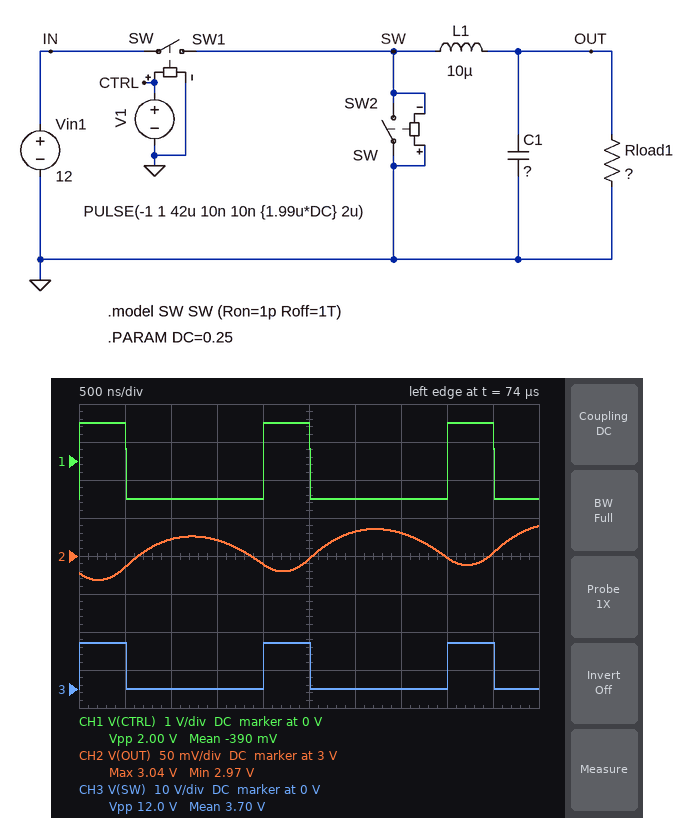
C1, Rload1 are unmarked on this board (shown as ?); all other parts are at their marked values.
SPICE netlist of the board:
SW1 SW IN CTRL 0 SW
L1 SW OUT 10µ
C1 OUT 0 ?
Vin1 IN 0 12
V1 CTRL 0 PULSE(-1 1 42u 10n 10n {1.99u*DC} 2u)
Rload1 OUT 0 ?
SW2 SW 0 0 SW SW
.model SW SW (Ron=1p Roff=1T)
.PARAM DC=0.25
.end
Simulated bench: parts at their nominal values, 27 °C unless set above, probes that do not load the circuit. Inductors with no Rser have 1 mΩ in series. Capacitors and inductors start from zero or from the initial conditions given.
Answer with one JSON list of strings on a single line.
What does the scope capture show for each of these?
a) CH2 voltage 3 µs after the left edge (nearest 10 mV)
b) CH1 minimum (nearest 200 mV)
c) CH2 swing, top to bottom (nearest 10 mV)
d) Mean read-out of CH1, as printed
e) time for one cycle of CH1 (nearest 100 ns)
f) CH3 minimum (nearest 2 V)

["3.03 V", "-1.0 V", "70 mV", "-390 mV", "2.0 µs", "0 V"]
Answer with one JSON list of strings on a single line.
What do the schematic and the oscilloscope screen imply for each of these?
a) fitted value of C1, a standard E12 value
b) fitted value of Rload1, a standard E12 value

["2.2 µF", "1 Ω"]
